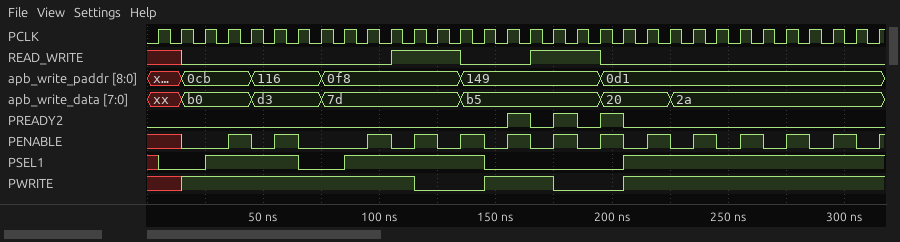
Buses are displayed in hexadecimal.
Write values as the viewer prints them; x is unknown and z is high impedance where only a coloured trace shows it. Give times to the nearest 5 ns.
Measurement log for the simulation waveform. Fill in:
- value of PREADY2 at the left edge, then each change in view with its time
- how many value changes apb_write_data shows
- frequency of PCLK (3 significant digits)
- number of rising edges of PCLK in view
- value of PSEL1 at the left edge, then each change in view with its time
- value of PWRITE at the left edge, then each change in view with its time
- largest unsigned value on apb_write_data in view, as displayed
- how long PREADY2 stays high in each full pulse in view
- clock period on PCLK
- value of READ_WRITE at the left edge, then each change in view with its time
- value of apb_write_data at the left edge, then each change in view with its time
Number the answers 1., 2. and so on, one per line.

1. 0, 1 at 155 ns, 0 at 165 ns, 1 at 175 ns, 0 at 185 ns, 1 at 195 ns, 0 at 205 ns
2. 6
3. 100 MHz
4. 32
5. x, 0 at 5 ns, 1 at 25 ns, 0 at 65 ns, 1 at 85 ns, 0 at 145 ns, 1 at 205 ns
6. x, 1 at 15 ns, 0 at 115 ns, 1 at 145 ns, 0 at 175 ns, 1 at 205 ns
7. d3
8. 10 ns, 10 ns, 10 ns
9. 10 ns
10. x, 0 at 15 ns, 1 at 105 ns, 0 at 135 ns, 1 at 165 ns, 0 at 195 ns
11. xx, b0 at 15 ns, d3 at 45 ns, 7d at 75 ns, b5 at 135 ns, 20 at 195 ns, 2a at 225 ns
